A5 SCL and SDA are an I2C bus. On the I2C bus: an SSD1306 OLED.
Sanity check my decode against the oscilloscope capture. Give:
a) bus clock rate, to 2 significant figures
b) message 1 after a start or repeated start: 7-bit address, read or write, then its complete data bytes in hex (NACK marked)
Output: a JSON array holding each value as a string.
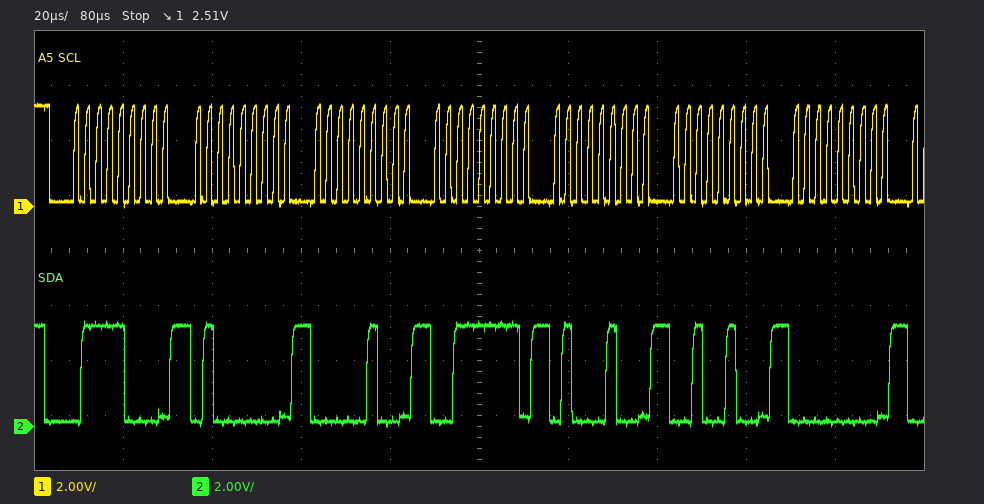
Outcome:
["400 kHz", "0x3C write: 40 04 3F 44 24 00"]
